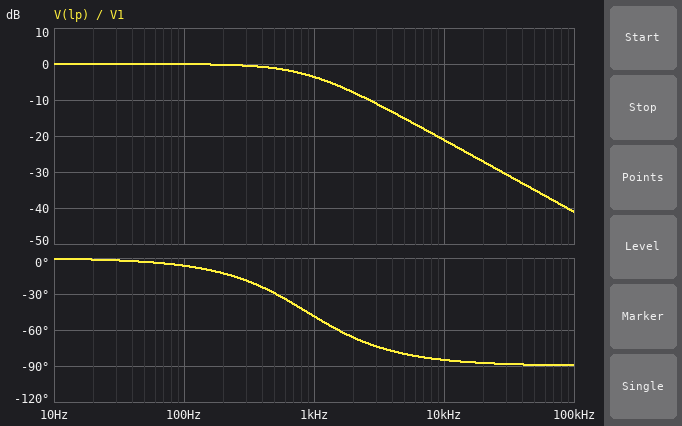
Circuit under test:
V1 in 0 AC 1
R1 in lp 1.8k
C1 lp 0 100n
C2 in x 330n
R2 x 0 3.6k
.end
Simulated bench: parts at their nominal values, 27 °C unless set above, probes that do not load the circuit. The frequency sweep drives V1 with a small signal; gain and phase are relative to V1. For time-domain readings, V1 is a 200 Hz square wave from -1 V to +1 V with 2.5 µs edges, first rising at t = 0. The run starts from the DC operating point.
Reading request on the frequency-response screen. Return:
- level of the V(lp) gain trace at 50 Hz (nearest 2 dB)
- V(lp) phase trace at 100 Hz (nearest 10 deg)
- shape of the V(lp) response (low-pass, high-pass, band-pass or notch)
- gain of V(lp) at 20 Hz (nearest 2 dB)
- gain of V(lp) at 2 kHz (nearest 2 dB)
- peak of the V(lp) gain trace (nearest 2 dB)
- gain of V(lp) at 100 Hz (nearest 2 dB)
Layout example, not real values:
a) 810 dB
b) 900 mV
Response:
a) 0 dB
b) -10 deg
c) low-pass
d) 0 dB
e) -8 dB
f) 0 dB
g) 0 dB
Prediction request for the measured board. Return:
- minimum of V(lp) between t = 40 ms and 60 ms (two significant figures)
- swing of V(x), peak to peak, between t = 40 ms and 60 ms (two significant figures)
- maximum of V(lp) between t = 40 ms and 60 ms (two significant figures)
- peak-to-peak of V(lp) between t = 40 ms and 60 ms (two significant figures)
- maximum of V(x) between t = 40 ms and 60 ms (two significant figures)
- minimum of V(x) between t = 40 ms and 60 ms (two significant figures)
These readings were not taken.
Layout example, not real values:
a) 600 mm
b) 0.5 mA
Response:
a) -1.0 V
b) 3.6 V
c) 1.0 V
d) 2.0 V
e) 1.8 V
f) -1.8 V
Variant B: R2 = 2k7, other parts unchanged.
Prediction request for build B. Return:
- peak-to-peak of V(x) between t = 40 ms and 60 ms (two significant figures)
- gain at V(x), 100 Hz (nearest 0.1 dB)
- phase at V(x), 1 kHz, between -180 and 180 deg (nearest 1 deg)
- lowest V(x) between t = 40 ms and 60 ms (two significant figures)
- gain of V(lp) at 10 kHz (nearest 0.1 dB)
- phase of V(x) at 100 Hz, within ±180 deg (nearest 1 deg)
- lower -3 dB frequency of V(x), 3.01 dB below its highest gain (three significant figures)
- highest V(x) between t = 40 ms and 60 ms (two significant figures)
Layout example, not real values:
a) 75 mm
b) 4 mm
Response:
a) 3.8 V
b) -6.2 dB
c) 10 deg
d) -1.9 V
e) -21.1 dB
f) 61 deg
g) 179 Hz
h) 1.9 V
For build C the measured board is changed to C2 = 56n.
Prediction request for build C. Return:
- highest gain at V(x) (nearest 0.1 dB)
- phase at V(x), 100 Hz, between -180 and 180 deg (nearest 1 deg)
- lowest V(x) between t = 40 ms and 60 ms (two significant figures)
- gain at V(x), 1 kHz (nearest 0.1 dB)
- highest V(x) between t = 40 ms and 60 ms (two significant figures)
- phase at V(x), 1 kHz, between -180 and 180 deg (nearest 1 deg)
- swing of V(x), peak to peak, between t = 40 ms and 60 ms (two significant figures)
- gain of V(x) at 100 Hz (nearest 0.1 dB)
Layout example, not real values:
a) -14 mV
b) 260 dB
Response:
a) 0 dB
b) 83 deg
c) -2.0 V
d) -2.1 dB
e) 2.0 V
f) 38 deg
g) 4.0 V
h) -18.0 dB
